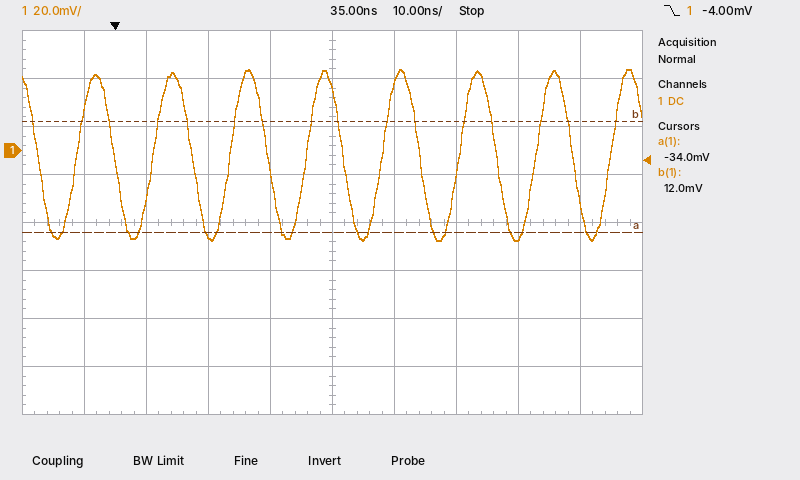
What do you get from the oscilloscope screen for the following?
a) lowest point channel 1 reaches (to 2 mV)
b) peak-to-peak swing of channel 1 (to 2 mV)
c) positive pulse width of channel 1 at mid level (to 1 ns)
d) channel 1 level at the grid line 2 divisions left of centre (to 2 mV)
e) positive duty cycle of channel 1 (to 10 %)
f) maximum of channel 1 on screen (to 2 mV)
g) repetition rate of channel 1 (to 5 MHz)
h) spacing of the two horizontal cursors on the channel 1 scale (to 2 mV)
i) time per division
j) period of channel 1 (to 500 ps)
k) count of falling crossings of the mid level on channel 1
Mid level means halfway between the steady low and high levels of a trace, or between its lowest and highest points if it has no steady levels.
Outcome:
-38 mV
72 mV
6 ns
-36 mV
50 %
34 mV
80 MHz
46 mV
10 ns
12.5 ns
8
